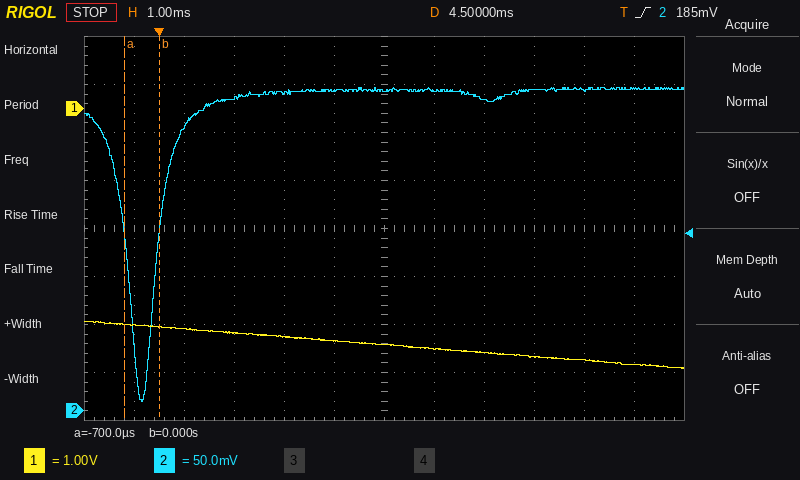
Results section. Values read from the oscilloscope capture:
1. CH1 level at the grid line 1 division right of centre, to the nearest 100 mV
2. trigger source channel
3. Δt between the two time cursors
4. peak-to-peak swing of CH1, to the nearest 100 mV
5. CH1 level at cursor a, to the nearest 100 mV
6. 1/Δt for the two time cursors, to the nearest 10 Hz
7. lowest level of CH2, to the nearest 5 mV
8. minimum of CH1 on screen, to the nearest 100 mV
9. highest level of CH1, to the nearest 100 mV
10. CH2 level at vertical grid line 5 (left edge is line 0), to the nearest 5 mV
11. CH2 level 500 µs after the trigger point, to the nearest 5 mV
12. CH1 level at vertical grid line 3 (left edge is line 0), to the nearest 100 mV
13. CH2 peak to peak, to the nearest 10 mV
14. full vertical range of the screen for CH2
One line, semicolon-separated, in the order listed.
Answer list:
-5.0 V; CH2; 700 µs; 1.0 V; -4.5 V; 1.43 kHz; 10 mV; -5.4 V; -4.4 V; 335 mV; 295 mV; -4.7 V; 330 mV; 400 mV
